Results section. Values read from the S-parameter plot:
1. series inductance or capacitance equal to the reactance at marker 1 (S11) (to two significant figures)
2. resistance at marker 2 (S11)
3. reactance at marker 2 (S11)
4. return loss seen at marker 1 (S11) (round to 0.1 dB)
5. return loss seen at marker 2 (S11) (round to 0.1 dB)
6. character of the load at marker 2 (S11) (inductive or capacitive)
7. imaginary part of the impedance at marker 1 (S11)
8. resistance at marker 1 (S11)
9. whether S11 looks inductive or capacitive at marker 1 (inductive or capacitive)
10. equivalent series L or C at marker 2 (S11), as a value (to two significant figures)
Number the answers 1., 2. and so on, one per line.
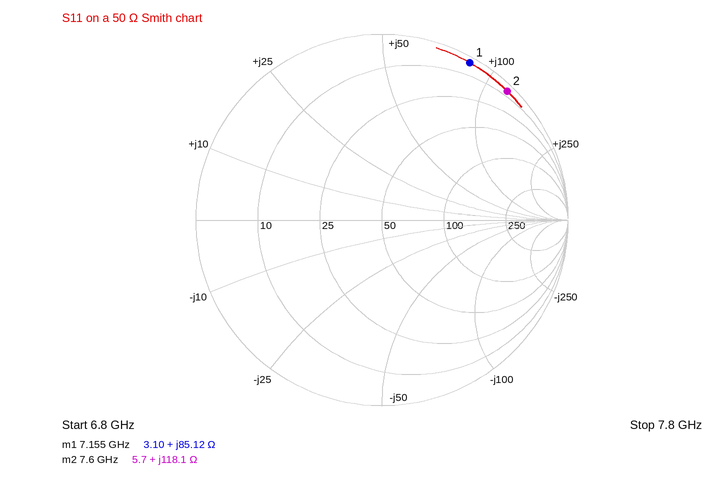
1. 1.9 nH
2. 5.7 Ω
3. +118.1 Ω
4. 0.3 dB
5. 0.3 dB
6. inductive
7. +85.12 Ω
8. 3.10 Ω
9. inductive
10. 2.5 nH
